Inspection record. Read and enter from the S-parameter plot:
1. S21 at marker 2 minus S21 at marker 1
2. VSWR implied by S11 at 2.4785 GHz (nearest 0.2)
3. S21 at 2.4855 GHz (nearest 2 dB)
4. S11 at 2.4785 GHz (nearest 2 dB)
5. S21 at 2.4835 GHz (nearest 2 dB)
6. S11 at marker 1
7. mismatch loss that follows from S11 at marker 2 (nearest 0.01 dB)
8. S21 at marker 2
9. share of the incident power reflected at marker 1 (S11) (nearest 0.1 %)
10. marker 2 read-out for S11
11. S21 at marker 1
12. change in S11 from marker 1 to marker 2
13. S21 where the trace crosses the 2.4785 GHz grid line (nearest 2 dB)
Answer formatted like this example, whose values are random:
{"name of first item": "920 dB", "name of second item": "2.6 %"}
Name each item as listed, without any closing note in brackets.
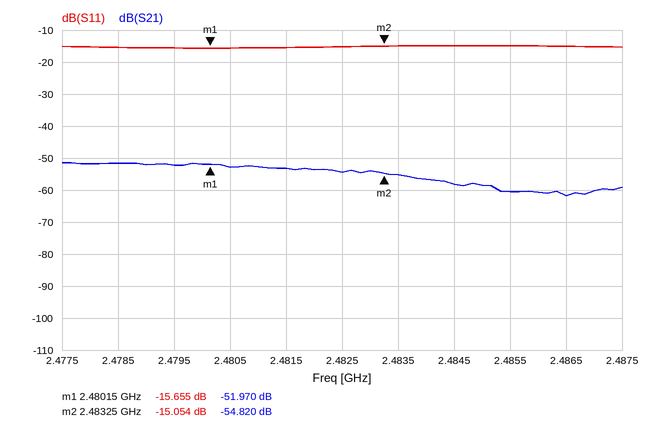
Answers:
{"S21 at marker 2 minus S21 at marker 1": "-2.850 dB", "VSWR implied by S11 at 2.4785 GHz": "1.4", "S21 at 2.4855 GHz": "-60 dB", "S11 at 2.4785 GHz": "-16 dB", "S21 at 2.4835 GHz": "-56 dB", "S11 at marker 1": "-15.655 dB", "mismatch loss that follows from S11 at marker 2": "0.14 dB", "S21 at marker 2": "-54.820 dB", "share of the incident power reflected at marker 1 (S11)": "2.7 %", "marker 2 read-out for S11": "-15.054 dB", "S21 at marker 1": "-51.970 dB", "change in S11 from marker 1 to marker 2": "0.601 dB", "S21 where the trace crosses the 2.4785 GHz grid line": "-52 dB"}
